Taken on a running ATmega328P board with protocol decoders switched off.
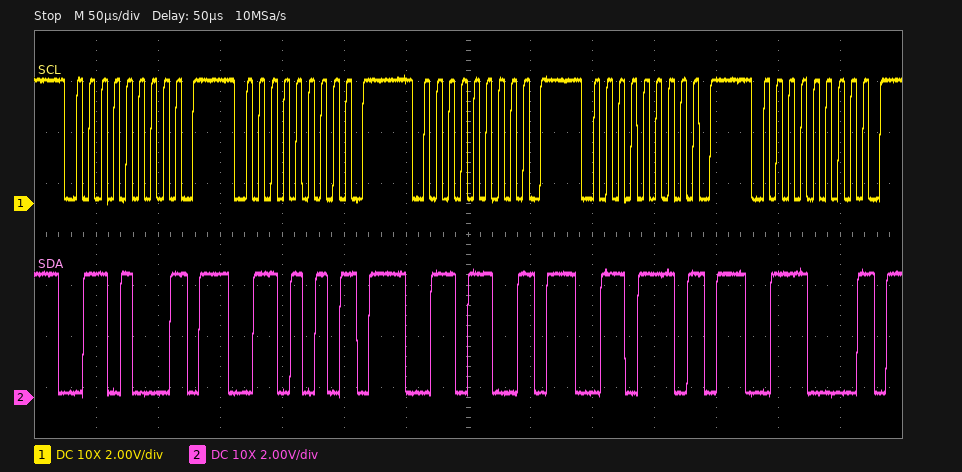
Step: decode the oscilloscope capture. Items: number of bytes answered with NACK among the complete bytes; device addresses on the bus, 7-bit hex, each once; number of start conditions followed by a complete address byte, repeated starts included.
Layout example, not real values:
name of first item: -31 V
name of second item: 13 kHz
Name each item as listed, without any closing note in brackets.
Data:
number of bytes answered with NACK among the complete bytes: 5
device addresses on the bus, 7-bit hex, each once: 0x34 0x35 0x36 0x37 0x38
number of start conditions followed by a complete address byte, repeated starts included: 5
